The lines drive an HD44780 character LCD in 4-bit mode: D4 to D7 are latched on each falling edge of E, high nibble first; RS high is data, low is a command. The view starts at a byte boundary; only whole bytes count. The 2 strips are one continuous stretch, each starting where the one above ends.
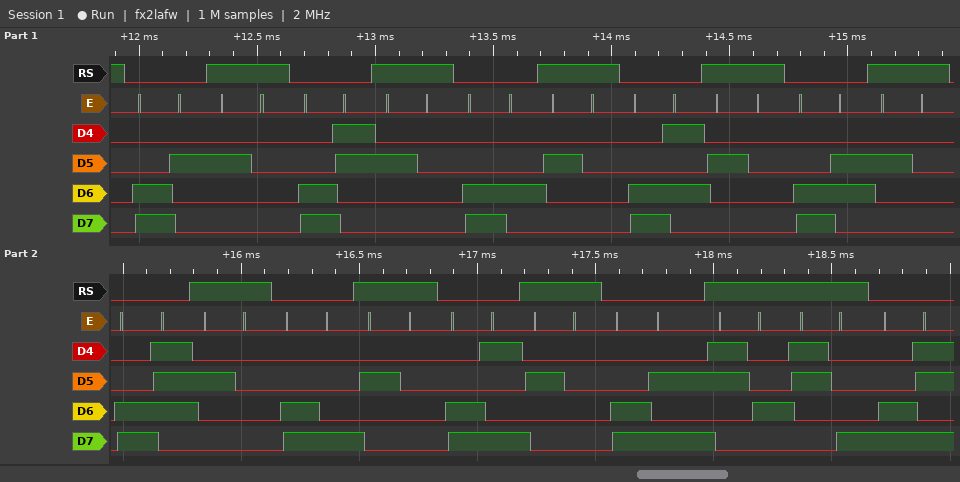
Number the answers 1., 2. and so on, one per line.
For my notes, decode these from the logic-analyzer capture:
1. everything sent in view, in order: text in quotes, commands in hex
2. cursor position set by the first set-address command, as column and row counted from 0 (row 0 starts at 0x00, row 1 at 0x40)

1. 0xC2 " " 0xC3 " " 0xC4 " " 0xC5 " " 0xC6 " " 0xC7 " " 0xC8 " " 0xC9 " " 0xCA "48" 0xCB
2. column 2, row 1
